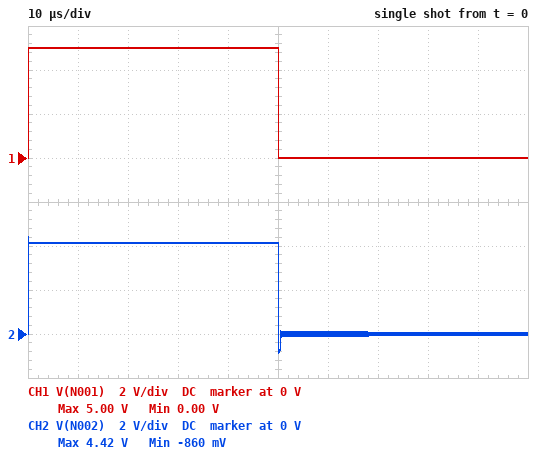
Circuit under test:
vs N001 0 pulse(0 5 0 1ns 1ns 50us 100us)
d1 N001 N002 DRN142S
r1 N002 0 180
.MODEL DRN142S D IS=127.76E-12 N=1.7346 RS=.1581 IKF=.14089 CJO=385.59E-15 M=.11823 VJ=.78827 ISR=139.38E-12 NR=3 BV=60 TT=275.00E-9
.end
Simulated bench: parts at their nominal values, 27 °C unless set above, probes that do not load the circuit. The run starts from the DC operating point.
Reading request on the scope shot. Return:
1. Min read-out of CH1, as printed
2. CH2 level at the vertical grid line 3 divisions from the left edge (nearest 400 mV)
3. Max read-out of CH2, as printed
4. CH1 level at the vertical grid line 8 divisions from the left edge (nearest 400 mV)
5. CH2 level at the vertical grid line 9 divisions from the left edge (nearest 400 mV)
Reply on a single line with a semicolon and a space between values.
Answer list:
0.00 V; 4.0 V; 4.42 V; 0 V; 0 V
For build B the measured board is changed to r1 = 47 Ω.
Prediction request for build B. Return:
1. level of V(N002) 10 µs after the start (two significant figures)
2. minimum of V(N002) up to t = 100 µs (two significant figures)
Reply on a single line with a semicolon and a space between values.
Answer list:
4.0 V; -940 mV
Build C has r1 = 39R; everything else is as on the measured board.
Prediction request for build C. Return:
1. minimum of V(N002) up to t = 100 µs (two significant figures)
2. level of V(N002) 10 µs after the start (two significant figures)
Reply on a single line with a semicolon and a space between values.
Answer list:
-950 mV; 4.0 V
